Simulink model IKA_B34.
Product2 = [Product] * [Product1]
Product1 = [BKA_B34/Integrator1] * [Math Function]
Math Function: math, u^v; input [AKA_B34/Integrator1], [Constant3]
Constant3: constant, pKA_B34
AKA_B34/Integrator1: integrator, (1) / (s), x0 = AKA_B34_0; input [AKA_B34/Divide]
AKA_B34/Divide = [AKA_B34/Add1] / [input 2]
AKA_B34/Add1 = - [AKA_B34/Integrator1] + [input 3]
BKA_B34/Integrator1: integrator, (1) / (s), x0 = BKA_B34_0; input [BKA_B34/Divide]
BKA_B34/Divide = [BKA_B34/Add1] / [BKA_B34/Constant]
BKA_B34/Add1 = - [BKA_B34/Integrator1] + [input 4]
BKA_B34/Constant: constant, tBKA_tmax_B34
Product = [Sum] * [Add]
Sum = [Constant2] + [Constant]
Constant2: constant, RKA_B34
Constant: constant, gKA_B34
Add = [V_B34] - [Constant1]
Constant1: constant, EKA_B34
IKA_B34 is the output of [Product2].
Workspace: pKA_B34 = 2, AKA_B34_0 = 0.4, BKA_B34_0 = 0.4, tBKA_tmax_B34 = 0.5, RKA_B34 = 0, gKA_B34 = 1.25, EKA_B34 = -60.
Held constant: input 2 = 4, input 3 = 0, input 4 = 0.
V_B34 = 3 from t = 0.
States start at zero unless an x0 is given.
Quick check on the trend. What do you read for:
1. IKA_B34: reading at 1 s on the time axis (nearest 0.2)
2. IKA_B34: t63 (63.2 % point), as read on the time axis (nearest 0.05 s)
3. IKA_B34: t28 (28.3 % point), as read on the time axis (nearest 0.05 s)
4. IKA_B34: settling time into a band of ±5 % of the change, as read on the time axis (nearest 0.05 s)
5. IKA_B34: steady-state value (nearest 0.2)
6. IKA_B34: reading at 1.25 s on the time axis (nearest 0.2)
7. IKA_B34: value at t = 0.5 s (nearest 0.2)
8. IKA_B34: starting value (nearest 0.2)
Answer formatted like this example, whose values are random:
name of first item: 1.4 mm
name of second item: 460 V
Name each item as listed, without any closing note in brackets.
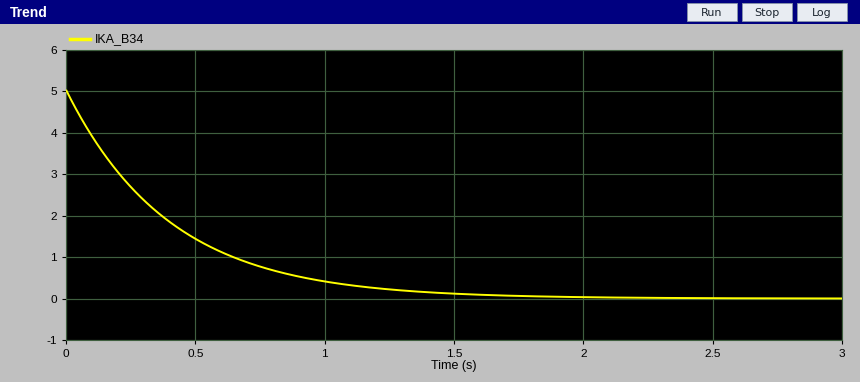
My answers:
IKA_B34: reading at 1 s on the time axis: 0.4
IKA_B34: t63 (63.2 % point), as read on the time axis: 0.40 s
IKA_B34: t28 (28.3 % point), as read on the time axis: 0.15 s
IKA_B34: settling time into a band of ±5 % of the change, as read on the time axis: 1.20 s
IKA_B34: steady-state value: 0.0
IKA_B34: reading at 1.25 s on the time axis: 0.2
IKA_B34: value at t = 0.5 s: 1.4
IKA_B34: starting value: 5.0
